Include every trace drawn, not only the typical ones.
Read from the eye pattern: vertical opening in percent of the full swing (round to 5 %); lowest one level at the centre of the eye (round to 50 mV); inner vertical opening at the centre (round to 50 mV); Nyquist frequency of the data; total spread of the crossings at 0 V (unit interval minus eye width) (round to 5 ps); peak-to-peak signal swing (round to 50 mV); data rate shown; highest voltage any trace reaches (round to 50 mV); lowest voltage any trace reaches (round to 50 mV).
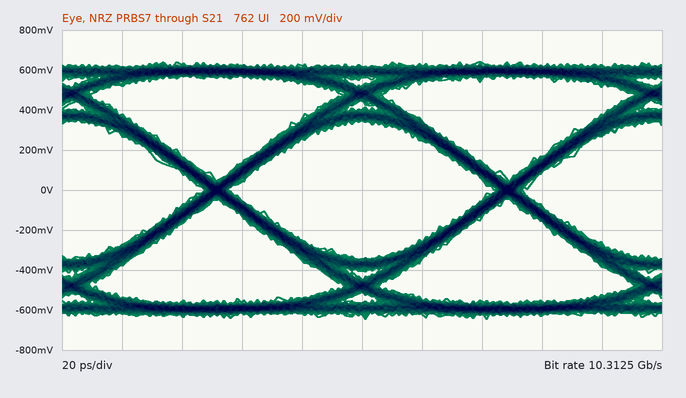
55 %
350 mV
700 mV
5.15625 GHz
10 ps
1.30 V
10.3125 Gb/s
650 mV
-650 mV
